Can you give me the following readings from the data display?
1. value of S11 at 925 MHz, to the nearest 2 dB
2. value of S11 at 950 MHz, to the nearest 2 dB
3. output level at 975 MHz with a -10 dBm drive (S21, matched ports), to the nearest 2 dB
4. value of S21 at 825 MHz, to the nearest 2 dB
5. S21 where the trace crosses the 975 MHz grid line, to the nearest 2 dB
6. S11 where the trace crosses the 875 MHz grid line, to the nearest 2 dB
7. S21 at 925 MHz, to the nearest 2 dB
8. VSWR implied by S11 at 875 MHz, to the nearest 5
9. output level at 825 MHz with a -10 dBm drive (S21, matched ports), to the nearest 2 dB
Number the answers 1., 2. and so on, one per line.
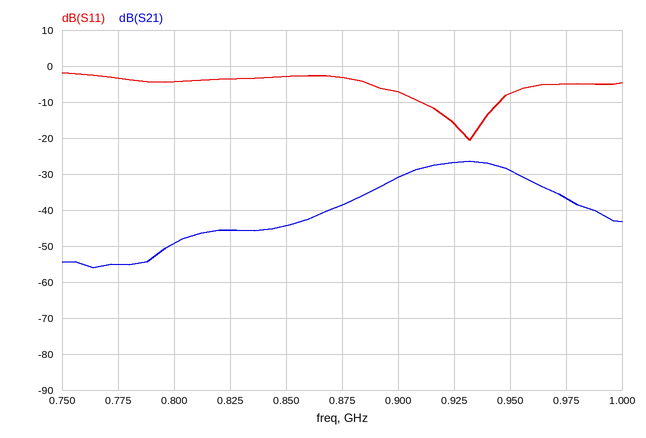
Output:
1. -16 dB
2. -8 dB
3. -46 dBm
4. -46 dB
5. -36 dB
6. -4 dB
7. -26 dB
8. 5
9. -56 dBm
